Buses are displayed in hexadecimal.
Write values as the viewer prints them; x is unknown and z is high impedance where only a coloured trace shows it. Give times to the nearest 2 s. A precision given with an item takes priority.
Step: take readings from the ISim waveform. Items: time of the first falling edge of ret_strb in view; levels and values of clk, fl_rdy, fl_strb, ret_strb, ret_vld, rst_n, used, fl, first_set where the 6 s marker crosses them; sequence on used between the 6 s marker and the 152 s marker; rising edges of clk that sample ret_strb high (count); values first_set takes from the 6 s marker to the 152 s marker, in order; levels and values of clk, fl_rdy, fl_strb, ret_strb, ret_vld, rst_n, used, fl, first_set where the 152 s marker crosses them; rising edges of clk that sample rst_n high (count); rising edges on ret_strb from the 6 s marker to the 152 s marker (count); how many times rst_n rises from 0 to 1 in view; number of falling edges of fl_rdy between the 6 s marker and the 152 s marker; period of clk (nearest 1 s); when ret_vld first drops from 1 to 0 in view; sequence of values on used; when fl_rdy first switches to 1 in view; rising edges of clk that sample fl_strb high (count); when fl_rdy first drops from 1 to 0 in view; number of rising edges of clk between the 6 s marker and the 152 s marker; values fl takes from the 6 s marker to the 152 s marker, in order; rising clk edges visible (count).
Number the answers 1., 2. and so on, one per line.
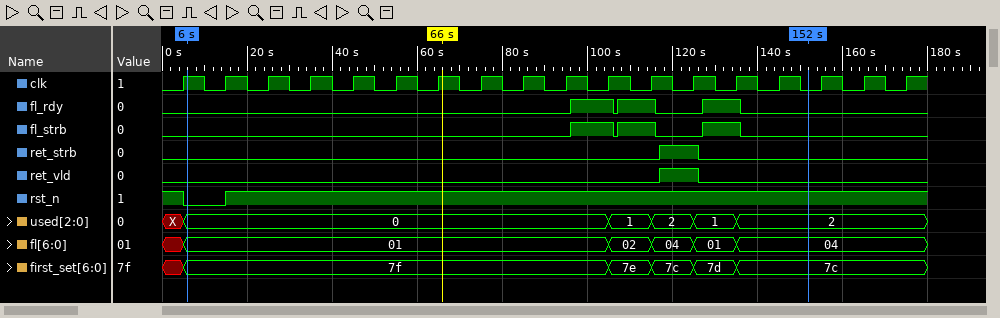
1. 126 s
2. clk=1, fl_rdy=0, fl_strb=0, ret_strb=0, ret_vld=0, rst_n=0, used=0, fl=01, first_set=7f
3. 0, 1, 2, 1, 2
4. 1
5. 7f, 7e, 7c, 7d, 7c
6. clk=0, fl_rdy=0, fl_strb=0, ret_strb=0, ret_vld=0, rst_n=1, used=2, fl=04, first_set=7c
7. 17
8. 1
9. 1
10. 3
11. 10 s
12. 126 s
13. X, 0, 1, 2, 1, 2
14. 96 s
15. 3
16. 106 s
17. 14
18. 01, 02, 04, 01, 04
19. 18
